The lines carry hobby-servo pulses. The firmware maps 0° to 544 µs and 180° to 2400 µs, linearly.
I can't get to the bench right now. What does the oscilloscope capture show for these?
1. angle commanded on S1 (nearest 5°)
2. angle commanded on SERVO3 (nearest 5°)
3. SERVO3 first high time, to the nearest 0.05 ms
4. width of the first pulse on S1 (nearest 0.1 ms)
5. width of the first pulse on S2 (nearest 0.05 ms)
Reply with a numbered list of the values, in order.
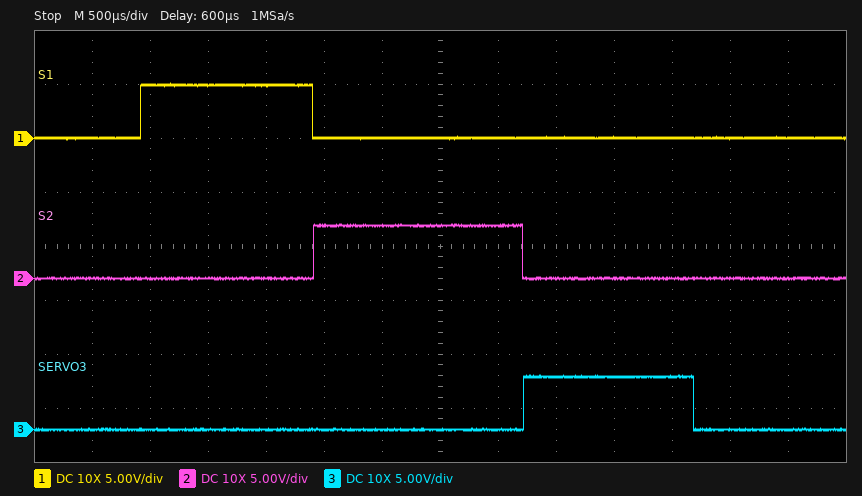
1. 90°
2. 90°
3. 1.45 ms
4. 1.5 ms
5. 1.80 ms
